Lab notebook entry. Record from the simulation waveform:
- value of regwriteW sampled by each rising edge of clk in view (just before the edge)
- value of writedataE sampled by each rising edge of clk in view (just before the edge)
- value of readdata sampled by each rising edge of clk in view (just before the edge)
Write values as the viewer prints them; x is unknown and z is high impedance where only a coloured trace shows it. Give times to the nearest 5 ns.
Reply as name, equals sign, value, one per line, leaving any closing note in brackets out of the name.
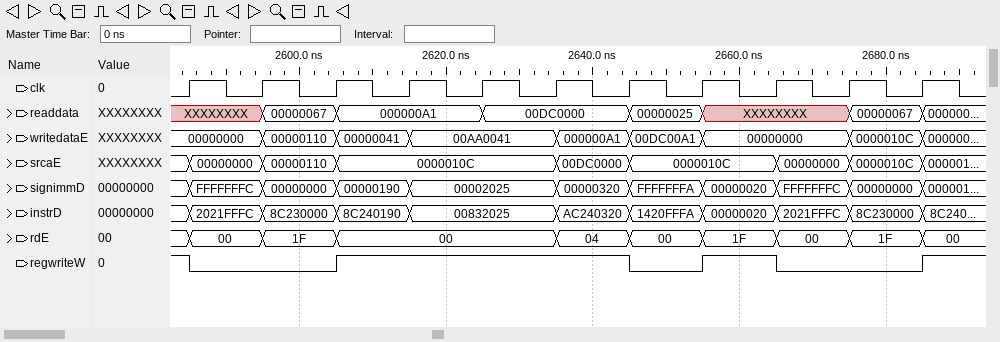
value of regwriteW sampled by each rising edge of clk in view = 1 0 0 1 1 1 1 0 1 0 0
value of writedataE sampled by each rising edge of clk in view = 00000000, 00000000, 00000110, 00000041, 00AA0041, 00AA0041, 000000A1, 00DC00A1, 00000000, 00000000, 0000010C
value of readdata sampled by each rising edge of clk in view = XXXXXXXX, XXXXXXXX, 00000067, 000000A1, 000000A1, 00DC0000, 00DC0000, 00000025, XXXXXXXX, XXXXXXXX, 00000067
